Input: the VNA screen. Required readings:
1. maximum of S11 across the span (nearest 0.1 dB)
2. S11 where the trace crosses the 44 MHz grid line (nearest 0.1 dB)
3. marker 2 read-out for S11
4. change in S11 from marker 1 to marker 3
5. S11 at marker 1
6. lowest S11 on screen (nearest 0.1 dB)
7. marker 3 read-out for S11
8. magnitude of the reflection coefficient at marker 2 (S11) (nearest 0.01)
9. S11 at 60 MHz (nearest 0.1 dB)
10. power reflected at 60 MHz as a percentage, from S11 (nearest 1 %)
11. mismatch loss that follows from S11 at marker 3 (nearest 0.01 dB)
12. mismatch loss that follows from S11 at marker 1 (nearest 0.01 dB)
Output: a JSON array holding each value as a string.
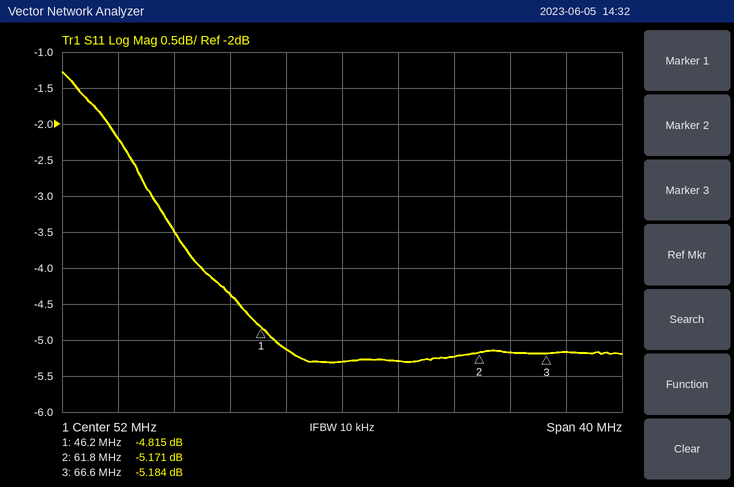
["-1.3 dB", "-4.4 dB", "-5.171 dB", "-0.369 dB", "-4.815 dB", "-5.3 dB", "-5.184 dB", "0.55", "-5.2 dB", "30 %", "1.57 dB", "1.74 dB"]
